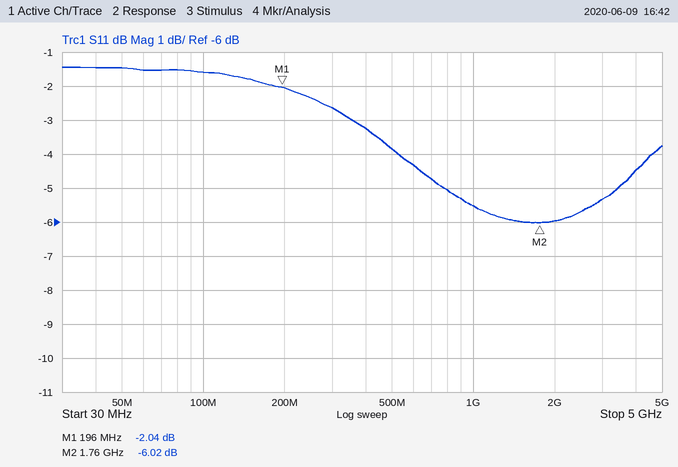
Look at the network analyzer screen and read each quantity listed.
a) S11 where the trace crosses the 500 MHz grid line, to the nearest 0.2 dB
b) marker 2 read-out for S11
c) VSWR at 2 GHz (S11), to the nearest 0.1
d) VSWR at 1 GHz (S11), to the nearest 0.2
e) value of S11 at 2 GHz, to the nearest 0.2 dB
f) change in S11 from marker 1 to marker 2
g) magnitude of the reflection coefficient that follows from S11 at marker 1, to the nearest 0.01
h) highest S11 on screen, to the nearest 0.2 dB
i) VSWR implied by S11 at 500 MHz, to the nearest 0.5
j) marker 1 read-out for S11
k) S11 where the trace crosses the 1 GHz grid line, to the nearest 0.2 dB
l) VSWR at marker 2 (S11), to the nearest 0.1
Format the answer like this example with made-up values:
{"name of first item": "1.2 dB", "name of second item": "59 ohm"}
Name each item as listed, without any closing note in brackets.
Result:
{"S11 where the trace crosses the 500 MHz grid line, to the nearest 0.2 dB": "-3.8 dB", "marker 2 read-out for S11": "-6.02 dB", "VSWR at 2 GHz (S11), to the nearest 0.1": "3.0", "VSWR at 1 GHz (S11), to the nearest 0.2": "3.2", "value of S11 at 2 GHz, to the nearest 0.2 dB": "-6.0 dB", "change in S11 from marker 1 to marker 2": "-3.98 dB", "magnitude of the reflection coefficient that follows from S11 at marker 1, to the nearest 0.01": "0.79", "highest S11 on screen, to the nearest 0.2 dB": "-1.4 dB", "VSWR implied by S11 at 500 MHz, to the nearest 0.5": "4.5", "marker 1 read-out for S11": "-2.04 dB", "S11 where the trace crosses the 1 GHz grid line, to the nearest 0.2 dB": "-5.6 dB", "VSWR at marker 2 (S11), to the nearest 0.1": "3.0"}
